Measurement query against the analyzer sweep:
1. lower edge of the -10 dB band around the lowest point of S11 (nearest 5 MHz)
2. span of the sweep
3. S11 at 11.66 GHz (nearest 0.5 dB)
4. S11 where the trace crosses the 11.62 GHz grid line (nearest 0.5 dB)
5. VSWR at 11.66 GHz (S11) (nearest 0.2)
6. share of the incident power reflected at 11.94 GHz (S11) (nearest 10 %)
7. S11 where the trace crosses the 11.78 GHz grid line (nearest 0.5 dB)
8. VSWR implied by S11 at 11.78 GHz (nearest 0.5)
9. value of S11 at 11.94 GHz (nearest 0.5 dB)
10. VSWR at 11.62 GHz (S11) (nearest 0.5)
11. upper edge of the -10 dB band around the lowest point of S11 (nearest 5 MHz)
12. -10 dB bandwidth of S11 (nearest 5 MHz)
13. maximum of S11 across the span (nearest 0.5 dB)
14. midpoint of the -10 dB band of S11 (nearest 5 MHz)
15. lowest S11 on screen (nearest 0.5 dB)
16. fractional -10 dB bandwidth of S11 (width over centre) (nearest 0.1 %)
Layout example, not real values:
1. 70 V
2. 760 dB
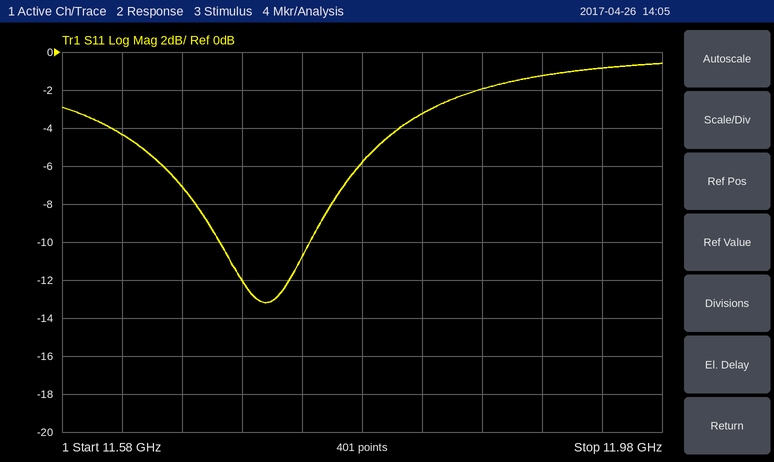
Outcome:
1. 11.685 GHz
2. 400 MHz
3. -7.0 dB
4. -4.5 dB
5. 2.6
6. 80 %
7. -6.0 dB
8. 3.0
9. -1.0 dB
10. 4.0
11. 11.745 GHz
12. 60 MHz
13. -0.5 dB
14. 11.715 GHz
15. -13.0 dB
16. 0.5 %
